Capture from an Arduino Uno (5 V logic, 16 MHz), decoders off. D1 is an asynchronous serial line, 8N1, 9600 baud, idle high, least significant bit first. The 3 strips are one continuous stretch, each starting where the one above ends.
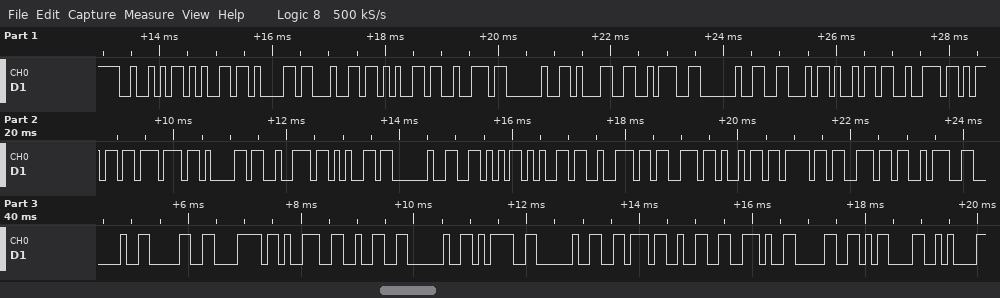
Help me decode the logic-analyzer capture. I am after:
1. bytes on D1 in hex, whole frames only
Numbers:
52 65 61 64 65 72 20 31 3A 20 46 69 72 6D 77 61 72 65 20 56 65 72 73 69 6F 6E 3A 20 30 78 39 32 20 3D 20 76 32 2E 30 0D 0A
